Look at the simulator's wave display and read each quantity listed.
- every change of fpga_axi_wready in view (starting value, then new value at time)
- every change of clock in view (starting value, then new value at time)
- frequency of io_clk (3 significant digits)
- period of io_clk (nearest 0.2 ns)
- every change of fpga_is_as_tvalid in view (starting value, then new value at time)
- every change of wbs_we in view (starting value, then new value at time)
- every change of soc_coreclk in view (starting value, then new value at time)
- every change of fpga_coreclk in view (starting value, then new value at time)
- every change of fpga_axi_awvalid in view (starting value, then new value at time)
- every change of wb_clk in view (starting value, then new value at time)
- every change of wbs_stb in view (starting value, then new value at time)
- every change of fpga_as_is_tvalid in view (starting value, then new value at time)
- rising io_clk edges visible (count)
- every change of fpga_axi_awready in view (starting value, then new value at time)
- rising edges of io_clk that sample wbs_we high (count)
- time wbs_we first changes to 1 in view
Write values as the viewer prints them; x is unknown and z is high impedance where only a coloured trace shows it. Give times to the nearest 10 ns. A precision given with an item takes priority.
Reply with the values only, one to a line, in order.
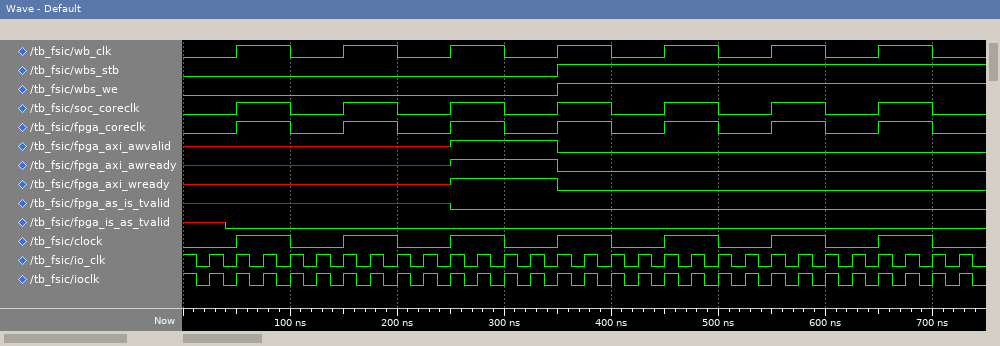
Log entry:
x, 1 at 250 ns, 0 at 350 ns
0, 1 at 50 ns, 0 at 100 ns, 1 at 150 ns, 0 at 200 ns, 1 at 250 ns, 0 at 300 ns, 1 at 350 ns, 0 at 400 ns, 1 at 450 ns, 0 at 500 ns, 1 at 550 ns, 0 at 600 ns, 1 at 650 ns, 0 at 700 ns
40.0 MHz
25 ns
x, 0 at 40 ns
0, 1 at 350 ns
0, 1 at 50 ns, 0 at 100 ns, 1 at 150 ns, 0 at 200 ns, 1 at 250 ns, 0 at 300 ns, 1 at 350 ns, 0 at 400 ns, 1 at 450 ns, 0 at 500 ns, 1 at 550 ns, 0 at 600 ns, 1 at 650 ns, 0 at 700 ns
0, 1 at 50 ns, 0 at 100 ns, 1 at 150 ns, 0 at 200 ns, 1 at 250 ns, 0 at 300 ns, 1 at 350 ns, 0 at 400 ns, 1 at 450 ns, 0 at 500 ns, 1 at 550 ns, 0 at 600 ns, 1 at 650 ns, 0 at 700 ns
x, 1 at 250 ns, 0 at 350 ns
0, 1 at 50 ns, 0 at 100 ns, 1 at 150 ns, 0 at 200 ns, 1 at 250 ns, 0 at 300 ns, 1 at 350 ns, 0 at 400 ns, 1 at 450 ns, 0 at 500 ns, 1 at 550 ns, 0 at 600 ns, 1 at 650 ns, 0 at 700 ns
0, 1 at 350 ns
x, 0 at 250 ns
29
x, 1 at 250 ns, 0 at 350 ns
15
350 ns
